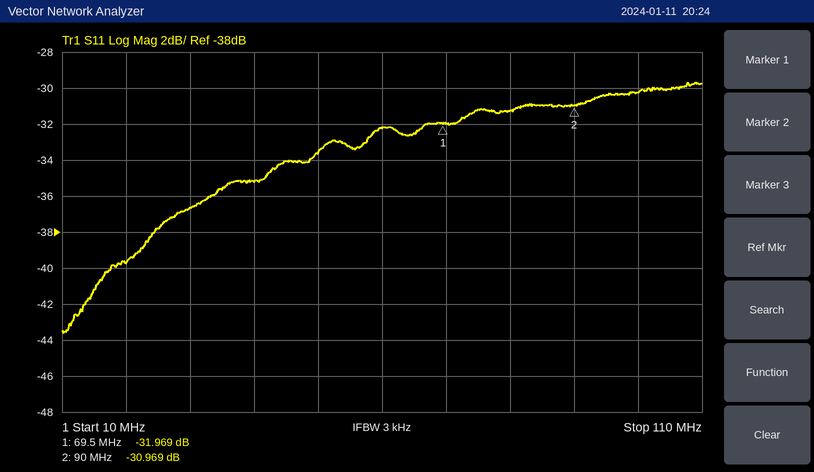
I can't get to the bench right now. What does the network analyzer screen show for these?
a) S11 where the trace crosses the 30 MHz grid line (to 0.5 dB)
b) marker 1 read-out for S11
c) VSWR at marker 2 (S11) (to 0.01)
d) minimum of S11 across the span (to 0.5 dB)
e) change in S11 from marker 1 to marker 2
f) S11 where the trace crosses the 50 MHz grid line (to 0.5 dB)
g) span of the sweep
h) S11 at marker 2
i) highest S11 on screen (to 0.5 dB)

-36.5 dB
-31.969 dB
1.06
-43.5 dB
1.000 dB
-33.5 dB
100 MHz
-30.969 dB
-29.5 dB
